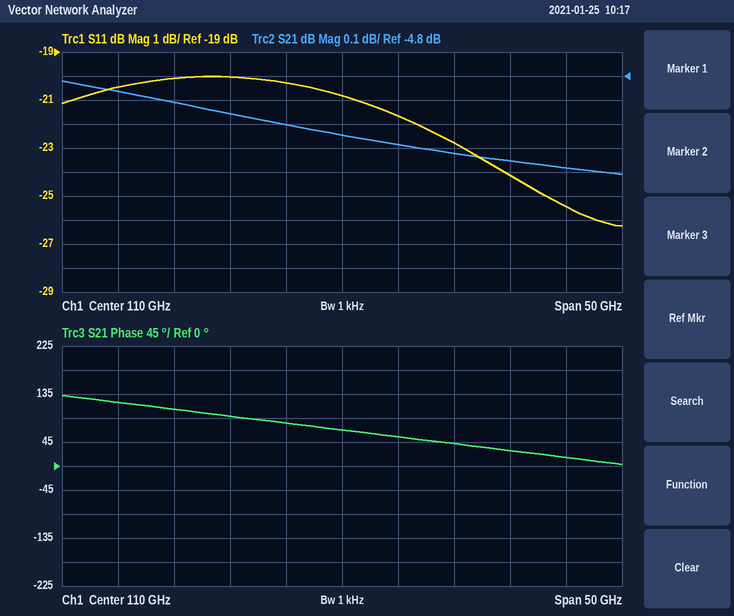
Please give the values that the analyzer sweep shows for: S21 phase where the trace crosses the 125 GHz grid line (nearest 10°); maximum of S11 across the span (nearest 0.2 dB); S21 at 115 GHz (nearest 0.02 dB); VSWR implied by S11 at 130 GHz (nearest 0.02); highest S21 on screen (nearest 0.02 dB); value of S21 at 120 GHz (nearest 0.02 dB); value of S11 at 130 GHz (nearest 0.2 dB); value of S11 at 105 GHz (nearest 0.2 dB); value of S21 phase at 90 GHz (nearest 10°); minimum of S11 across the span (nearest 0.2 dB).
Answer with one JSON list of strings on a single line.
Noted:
["30°", "-20.0 dB", "-5.08 dB", "1.12", "-4.82 dB", "-5.12 dB", "-25.4 dB", "-20.2 dB", "120°", "-26.2 dB"]
